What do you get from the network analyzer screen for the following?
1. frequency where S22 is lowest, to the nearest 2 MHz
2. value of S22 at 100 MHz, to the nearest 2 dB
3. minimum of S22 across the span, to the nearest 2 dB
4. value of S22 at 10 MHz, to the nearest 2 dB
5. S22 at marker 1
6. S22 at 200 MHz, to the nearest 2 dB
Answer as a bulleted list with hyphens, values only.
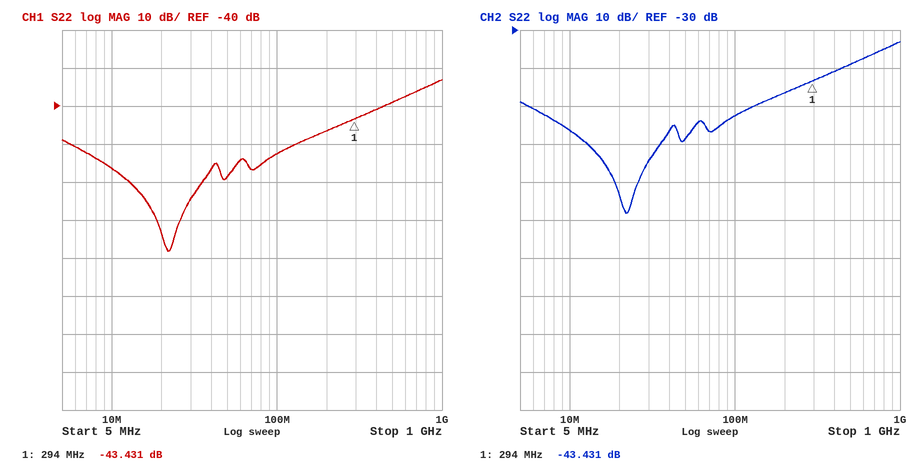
- 22 MHz
- -52 dB
- -78 dB
- -56 dB
- -43.431 dB
- -46 dB
